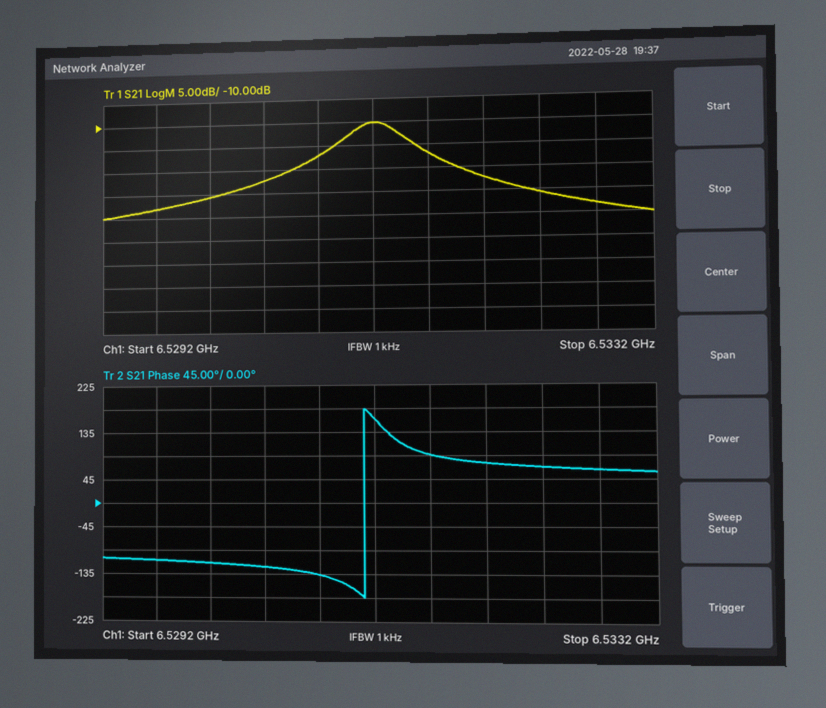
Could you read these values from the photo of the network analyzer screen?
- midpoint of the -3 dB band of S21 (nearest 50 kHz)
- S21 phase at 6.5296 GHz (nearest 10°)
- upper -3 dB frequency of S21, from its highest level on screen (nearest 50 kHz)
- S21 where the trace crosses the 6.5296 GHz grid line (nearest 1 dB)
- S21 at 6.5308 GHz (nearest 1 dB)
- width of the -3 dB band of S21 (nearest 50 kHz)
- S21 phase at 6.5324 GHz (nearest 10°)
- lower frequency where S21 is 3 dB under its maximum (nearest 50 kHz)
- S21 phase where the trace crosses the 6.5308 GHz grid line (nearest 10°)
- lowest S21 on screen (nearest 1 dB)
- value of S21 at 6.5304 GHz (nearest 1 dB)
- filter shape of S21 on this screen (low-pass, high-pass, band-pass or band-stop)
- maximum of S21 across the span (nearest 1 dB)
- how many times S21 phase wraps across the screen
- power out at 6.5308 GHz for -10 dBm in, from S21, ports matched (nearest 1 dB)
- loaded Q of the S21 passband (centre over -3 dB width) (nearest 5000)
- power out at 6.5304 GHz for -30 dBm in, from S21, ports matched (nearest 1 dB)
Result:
6.53120 GHz
-110°
6.53140 GHz
-28 dB
-17 dB
400 kHz
70°
6.53100 GHz
-140°
-30 dB
-22 dB
band-pass
-10 dB
1
-27 dBm
15000
-52 dBm
